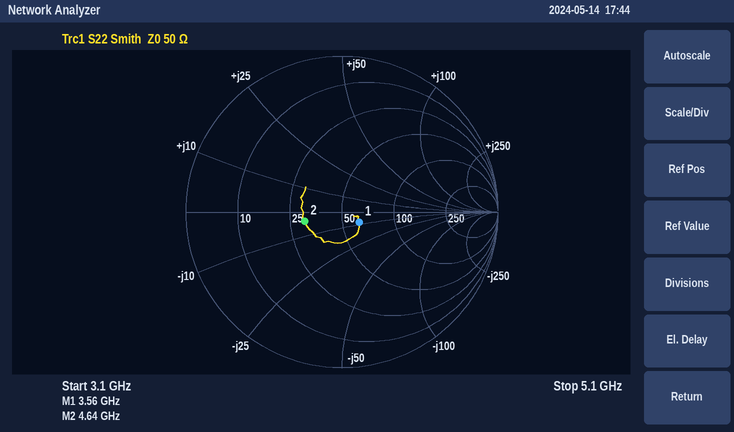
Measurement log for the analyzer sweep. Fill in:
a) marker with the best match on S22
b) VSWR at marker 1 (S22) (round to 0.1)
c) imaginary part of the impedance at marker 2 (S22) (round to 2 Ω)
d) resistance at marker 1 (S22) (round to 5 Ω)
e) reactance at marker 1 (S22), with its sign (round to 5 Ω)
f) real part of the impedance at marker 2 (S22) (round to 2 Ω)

marker 1
1.3
-4 Ω
60 Ω
-10 Ω
30 Ω
